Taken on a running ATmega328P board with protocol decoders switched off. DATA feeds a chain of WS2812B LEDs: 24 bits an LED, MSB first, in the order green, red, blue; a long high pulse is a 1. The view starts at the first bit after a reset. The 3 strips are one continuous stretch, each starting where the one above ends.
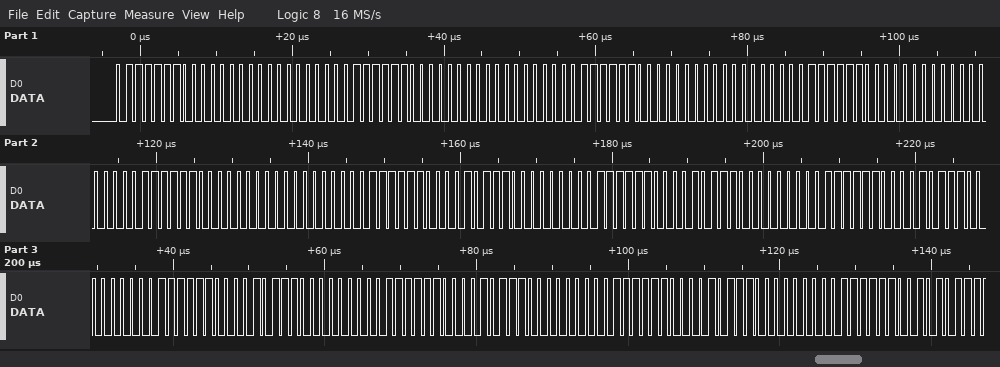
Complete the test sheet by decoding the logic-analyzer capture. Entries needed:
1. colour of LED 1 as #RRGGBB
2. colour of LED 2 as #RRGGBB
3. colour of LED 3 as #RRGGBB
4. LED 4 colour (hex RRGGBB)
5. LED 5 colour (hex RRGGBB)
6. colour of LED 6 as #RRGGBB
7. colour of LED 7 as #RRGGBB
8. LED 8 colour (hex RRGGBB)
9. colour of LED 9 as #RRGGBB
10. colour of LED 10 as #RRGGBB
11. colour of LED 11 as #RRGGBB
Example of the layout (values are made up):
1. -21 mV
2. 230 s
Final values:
1. #007E00
2. #007E00
3. #007E00
4. #007E00
5. #007E00
6. #177E00
7. #177E00
8. #177E00
9. #177E00
10. #177E00
11. #177E00
